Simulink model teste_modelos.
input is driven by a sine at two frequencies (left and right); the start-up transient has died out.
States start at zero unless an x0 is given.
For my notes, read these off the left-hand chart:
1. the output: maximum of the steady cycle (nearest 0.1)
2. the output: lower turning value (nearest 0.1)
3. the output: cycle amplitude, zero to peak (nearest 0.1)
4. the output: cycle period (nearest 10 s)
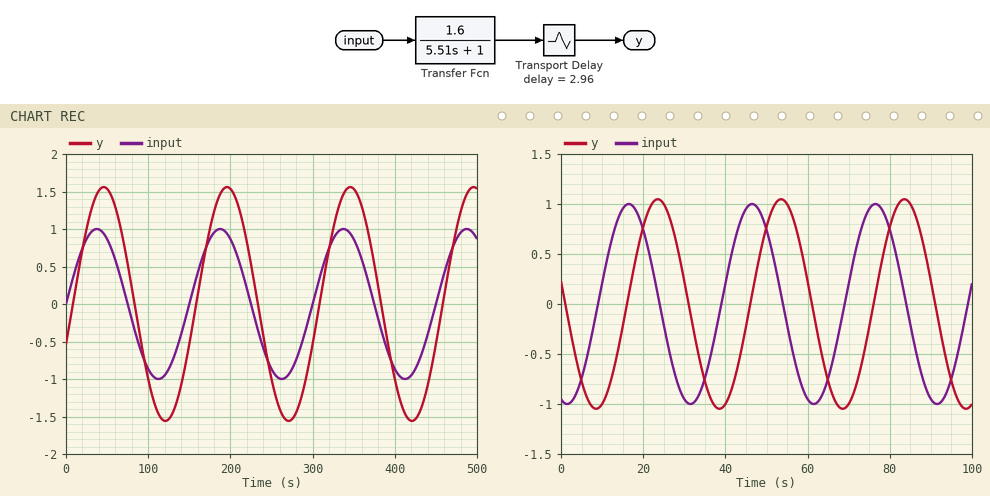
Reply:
1.6
-1.6
1.6
150 s
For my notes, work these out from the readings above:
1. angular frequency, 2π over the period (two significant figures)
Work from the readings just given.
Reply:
0.042 rad/s
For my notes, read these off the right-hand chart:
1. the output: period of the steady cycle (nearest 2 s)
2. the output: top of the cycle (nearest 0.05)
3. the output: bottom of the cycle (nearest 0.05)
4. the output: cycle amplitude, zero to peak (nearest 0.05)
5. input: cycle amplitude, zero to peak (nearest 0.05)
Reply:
30 s
1.05
-1.05
1.05
1.00
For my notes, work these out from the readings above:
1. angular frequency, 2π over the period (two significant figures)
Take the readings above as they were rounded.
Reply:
0.21 rad/s
